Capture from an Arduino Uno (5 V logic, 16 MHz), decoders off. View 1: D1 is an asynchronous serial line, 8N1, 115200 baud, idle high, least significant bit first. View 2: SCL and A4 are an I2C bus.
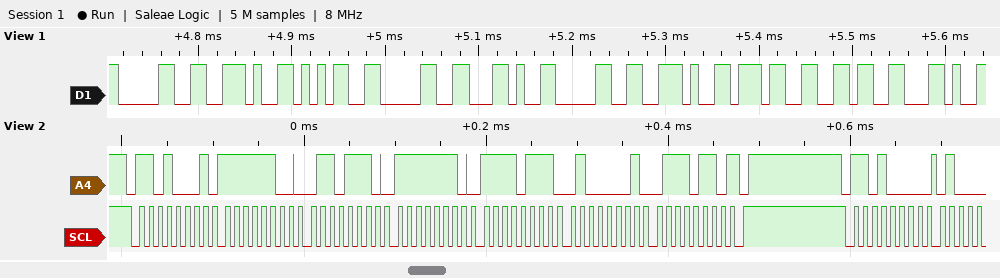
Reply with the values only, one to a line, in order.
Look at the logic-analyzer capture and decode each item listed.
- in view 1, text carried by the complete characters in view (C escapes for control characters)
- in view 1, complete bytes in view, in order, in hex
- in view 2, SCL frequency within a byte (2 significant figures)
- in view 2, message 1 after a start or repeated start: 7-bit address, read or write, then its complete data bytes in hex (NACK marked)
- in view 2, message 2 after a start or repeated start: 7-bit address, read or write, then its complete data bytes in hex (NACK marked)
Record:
"0.50,0.76,"
0x30 0x2E 0x35 0x30 0x2C 0x30 0x2E 0x37 0x36 0x2C
100 kHz
0x68 read: FC 6E FE F7 41 76 NACK
0x68 write
